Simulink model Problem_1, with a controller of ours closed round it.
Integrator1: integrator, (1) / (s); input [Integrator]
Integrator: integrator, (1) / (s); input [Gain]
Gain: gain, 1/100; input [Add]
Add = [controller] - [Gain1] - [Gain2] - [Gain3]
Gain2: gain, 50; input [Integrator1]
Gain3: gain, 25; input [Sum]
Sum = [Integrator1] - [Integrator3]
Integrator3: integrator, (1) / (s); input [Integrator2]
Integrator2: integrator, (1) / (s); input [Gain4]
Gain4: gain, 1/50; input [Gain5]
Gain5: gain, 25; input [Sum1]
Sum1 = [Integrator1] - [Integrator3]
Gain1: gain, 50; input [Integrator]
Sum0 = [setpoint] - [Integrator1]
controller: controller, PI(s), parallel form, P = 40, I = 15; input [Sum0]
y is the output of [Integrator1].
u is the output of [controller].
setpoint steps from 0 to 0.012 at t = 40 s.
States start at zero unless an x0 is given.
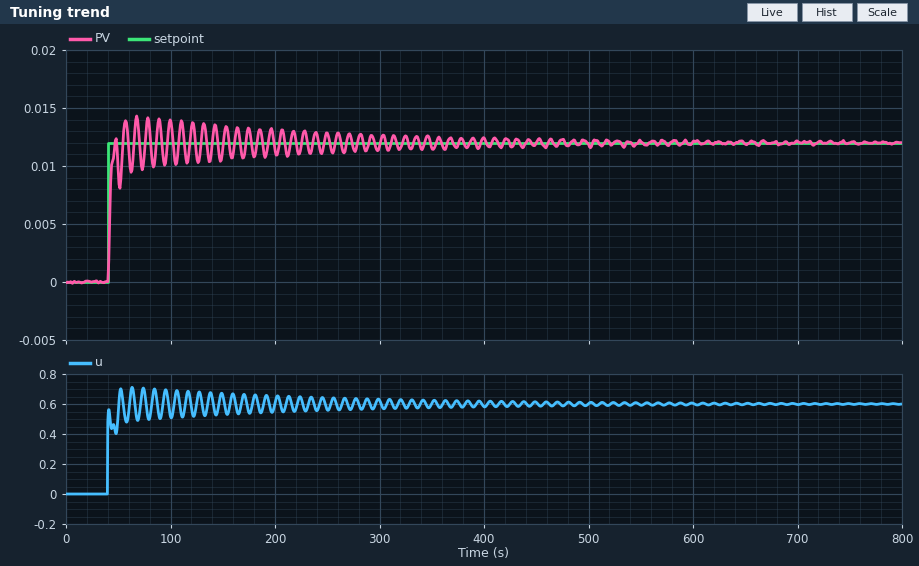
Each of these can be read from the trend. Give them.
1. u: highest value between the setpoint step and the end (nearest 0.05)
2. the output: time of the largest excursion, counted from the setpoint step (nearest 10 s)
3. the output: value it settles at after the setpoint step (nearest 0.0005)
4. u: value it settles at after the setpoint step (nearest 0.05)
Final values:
0.70
30 s
0.0120
0.60
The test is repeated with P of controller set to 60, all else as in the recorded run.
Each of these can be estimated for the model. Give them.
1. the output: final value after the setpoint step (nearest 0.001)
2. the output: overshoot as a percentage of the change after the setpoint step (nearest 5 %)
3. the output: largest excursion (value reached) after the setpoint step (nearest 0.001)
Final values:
0.012
15 %
0.014
